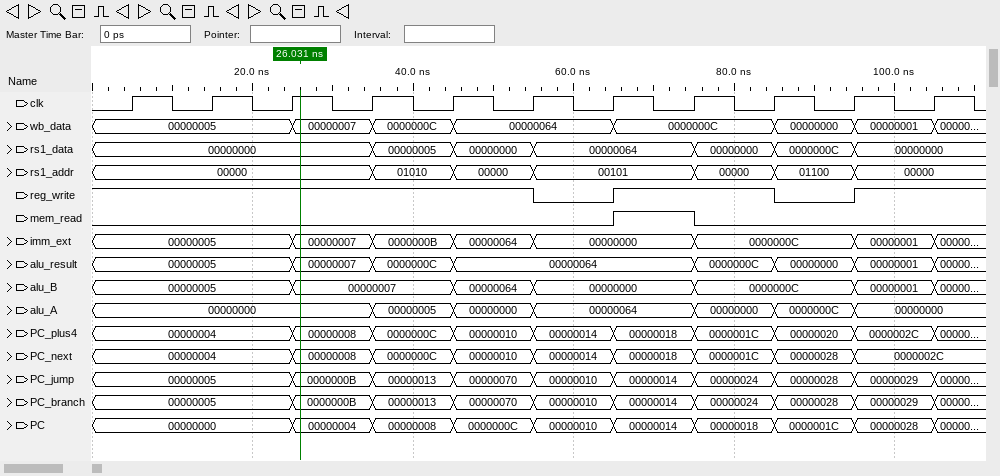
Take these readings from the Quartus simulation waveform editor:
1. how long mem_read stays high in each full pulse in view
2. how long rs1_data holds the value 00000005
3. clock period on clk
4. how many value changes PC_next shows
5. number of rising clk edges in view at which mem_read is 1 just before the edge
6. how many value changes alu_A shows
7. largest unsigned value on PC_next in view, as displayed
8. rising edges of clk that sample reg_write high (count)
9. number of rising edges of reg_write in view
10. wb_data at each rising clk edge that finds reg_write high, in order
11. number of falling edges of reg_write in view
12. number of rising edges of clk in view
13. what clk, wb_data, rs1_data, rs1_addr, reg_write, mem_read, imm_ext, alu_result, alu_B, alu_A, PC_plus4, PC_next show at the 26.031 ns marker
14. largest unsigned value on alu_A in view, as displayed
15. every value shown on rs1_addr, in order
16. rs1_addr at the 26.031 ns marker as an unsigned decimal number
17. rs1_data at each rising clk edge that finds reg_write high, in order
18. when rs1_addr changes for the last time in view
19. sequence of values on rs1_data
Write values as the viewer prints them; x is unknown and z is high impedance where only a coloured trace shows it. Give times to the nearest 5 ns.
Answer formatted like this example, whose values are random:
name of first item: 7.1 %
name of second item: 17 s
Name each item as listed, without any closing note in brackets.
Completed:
how long mem_read stays high in each full pulse in view: 10 ns
how long rs1_data holds the value 00000005: 10 ns
clock period on clk: 10 ns
how many value changes PC_next shows: 8
number of rising clk edges in view at which mem_read is 1 just before the edge: 1
how many value changes alu_A shows: 6
largest unsigned value on PC_next in view, as displayed: 0000002C
rising edges of clk that sample reg_write high: 9
number of rising edges of reg_write in view: 2
wb_data at each rising clk edge that finds reg_write high, in order: 00000005, 00000005, 00000005, 00000007, 0000000C, 00000064, 0000000C, 0000000C, 00000001
number of falling edges of reg_write in view: 2
number of rising edges of clk in view: 11
what clk, wb_data, rs1_data, rs1_addr, reg_write, mem_read, imm_ext, alu_result, alu_B, alu_A, PC_plus4, PC_next show at the 26.031 ns marker: clk=1, wb_data=00000007, rs1_data=00000000, rs1_addr=00000, reg_write=1, mem_read=0, imm_ext=00000007, alu_result=00000007, alu_B=00000007, alu_A=00000000, PC_plus4=00000008, PC_next=00000008
largest unsigned value on alu_A in view, as displayed: 00000064
every value shown on rs1_addr, in order: 00000, 01010, 00000, 00101, 00000, 01100, 00000
rs1_addr at the 26.031 ns marker as an unsigned decimal number: 0
rs1_data at each rising clk edge that finds reg_write high, in order: 00000000, 00000000, 00000000, 00000000, 00000005, 00000000, 00000064, 00000000, 00000000
when rs1_addr changes for the last time in view: 95 ns
sequence of values on rs1_data: 00000000, 00000005, 00000000, 00000064, 00000000, 0000000C, 00000000
